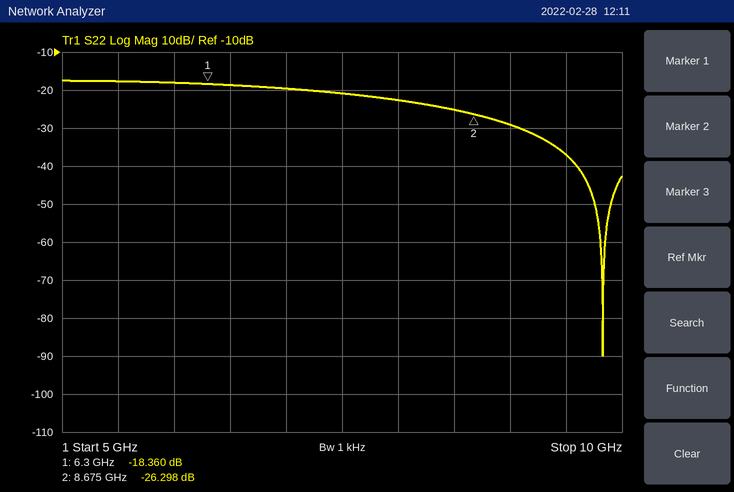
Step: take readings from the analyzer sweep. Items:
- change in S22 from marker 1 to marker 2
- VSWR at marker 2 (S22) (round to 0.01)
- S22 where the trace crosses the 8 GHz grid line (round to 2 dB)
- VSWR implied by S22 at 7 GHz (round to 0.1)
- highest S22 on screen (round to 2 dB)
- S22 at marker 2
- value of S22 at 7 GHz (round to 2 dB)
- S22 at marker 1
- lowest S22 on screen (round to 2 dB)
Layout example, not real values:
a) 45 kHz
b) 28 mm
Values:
a) -7.938 dB
b) 1.10
c) -22 dB
d) 1.2
e) -18 dB
f) -26.298 dB
g) -20 dB
h) -18.360 dB
i) -90 dB
